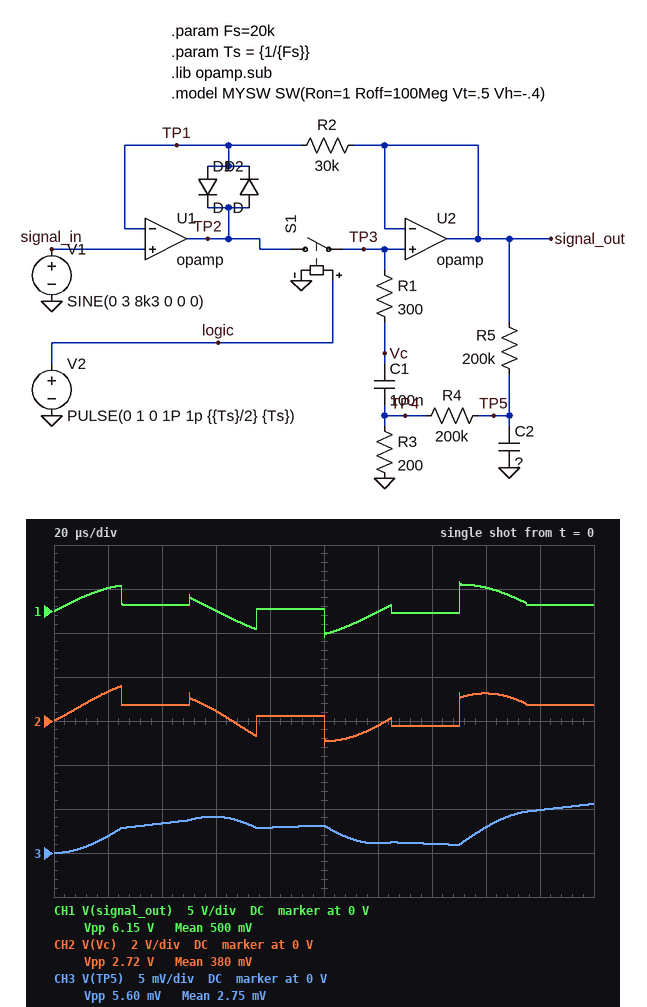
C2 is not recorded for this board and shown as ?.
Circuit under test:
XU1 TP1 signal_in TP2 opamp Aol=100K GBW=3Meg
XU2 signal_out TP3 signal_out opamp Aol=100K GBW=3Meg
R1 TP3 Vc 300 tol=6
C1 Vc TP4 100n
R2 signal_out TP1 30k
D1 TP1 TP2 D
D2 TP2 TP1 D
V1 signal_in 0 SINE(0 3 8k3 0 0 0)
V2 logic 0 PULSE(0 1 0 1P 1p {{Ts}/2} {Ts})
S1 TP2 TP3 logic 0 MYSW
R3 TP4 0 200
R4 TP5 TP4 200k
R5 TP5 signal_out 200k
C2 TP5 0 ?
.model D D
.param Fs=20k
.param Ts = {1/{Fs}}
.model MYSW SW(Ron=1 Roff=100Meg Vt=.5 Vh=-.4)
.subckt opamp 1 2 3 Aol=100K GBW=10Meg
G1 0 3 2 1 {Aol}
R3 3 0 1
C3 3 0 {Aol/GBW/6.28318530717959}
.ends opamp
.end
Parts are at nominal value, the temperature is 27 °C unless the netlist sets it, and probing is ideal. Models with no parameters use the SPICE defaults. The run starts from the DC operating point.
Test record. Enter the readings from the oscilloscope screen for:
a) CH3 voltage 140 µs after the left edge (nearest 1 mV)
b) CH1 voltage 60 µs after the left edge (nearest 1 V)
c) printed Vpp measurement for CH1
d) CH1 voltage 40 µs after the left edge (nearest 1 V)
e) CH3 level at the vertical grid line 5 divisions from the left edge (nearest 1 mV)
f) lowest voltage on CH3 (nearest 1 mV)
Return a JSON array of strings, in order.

["1 mV", "0 V", "6.15 V", "1 V", "3 mV", "0 V"]
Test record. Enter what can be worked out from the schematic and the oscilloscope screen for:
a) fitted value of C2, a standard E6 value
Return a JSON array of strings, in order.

["100 nF"]
